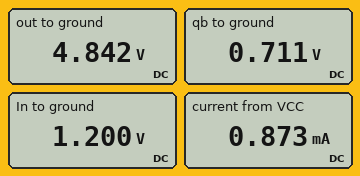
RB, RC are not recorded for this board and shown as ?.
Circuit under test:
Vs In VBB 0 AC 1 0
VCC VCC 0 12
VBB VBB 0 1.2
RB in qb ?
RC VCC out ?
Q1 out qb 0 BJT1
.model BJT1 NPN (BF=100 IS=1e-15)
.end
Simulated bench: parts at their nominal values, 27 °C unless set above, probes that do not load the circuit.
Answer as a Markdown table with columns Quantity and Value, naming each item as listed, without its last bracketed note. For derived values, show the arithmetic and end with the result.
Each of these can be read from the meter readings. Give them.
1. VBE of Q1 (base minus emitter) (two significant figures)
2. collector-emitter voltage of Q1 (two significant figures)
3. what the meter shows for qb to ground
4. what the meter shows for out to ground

| Quantity | Value |
|---|---|
| VBE of Q1 (base minus emitter) | 711 mV = 710 mV |
| collector-emitter voltage of Q1 | 4.842 V = 4.8 V |
| what the meter shows for qb to ground | 0.711 V |
| what the meter shows for out to ground | 4.842 V |
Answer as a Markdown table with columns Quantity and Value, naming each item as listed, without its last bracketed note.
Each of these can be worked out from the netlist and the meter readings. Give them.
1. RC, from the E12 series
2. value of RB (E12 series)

| Quantity | Value |
|---|---|
| RC, from the E12 series | 8.2 kΩ |
| value of RB | 56 kΩ |
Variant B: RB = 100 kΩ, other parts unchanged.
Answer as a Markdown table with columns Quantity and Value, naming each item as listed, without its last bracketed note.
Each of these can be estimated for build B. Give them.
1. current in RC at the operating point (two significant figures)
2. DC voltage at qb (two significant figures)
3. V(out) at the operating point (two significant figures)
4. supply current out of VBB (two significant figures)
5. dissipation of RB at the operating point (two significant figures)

| Quantity | Value |
|---|---|
| current in RC at the operating point | 500 µA |
| DC voltage at qb | 700 mV |
| V(out) at the operating point | 7.9 V |
| supply current out of VBB | 5.0 µA |
| dissipation of RB at the operating point | 2.5 µW |
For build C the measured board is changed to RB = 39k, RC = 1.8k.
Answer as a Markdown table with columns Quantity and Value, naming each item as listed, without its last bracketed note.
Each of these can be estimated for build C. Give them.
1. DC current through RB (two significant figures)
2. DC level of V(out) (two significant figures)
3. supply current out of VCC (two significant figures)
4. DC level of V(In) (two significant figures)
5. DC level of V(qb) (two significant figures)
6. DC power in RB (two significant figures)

| Quantity | Value |
|---|---|
| DC current through RB | 12 µA |
| DC level of V(out) | 9.8 V |
| supply current out of VCC | 1.2 mA |
| DC level of V(In) | 1.2 V |
| DC level of V(qb) | 720 mV |
| DC power in RB | 5.9 µW |
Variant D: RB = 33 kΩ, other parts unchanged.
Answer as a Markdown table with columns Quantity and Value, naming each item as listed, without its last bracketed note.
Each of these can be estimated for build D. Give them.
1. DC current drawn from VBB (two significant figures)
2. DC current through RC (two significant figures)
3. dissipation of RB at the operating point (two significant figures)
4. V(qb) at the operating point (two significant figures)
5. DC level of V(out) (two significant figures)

| Quantity | Value |
|---|---|
| DC current drawn from VBB | 14 µA |
| DC current through RC | 1.4 mA |
| dissipation of RB at the operating point | 6.9 µW |
| V(qb) at the operating point | 720 mV |
| DC level of V(out) | 250 mV |
